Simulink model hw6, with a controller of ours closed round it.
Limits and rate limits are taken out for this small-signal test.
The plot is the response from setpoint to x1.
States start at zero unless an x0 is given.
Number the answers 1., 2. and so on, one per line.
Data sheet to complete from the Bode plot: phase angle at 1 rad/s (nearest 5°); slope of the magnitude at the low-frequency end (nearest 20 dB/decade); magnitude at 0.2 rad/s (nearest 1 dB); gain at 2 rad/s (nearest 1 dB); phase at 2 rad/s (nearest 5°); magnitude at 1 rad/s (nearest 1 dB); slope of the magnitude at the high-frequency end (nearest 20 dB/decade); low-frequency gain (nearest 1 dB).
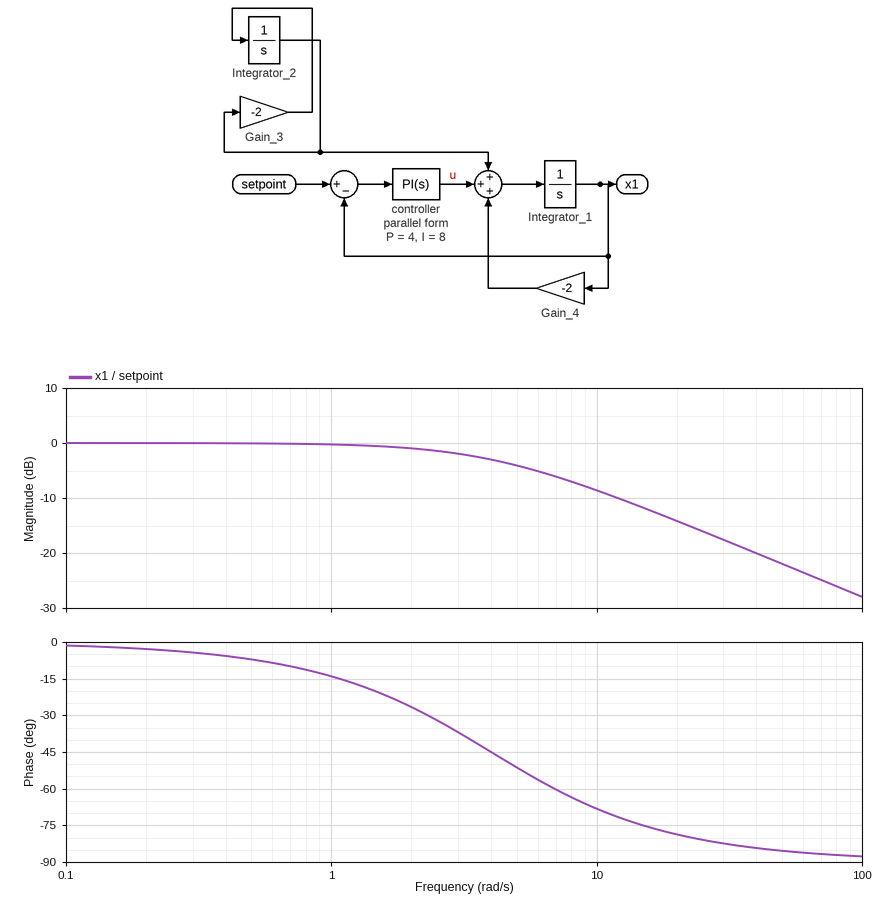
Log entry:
1. -15°
2. 0 dB/decade
3. 0 dB
4. -1 dB
5. -25°
6. 0 dB
7. -20 dB/decade
8. 0 dB
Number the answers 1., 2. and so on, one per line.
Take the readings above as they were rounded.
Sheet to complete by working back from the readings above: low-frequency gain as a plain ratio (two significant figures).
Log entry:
1. 1.0
